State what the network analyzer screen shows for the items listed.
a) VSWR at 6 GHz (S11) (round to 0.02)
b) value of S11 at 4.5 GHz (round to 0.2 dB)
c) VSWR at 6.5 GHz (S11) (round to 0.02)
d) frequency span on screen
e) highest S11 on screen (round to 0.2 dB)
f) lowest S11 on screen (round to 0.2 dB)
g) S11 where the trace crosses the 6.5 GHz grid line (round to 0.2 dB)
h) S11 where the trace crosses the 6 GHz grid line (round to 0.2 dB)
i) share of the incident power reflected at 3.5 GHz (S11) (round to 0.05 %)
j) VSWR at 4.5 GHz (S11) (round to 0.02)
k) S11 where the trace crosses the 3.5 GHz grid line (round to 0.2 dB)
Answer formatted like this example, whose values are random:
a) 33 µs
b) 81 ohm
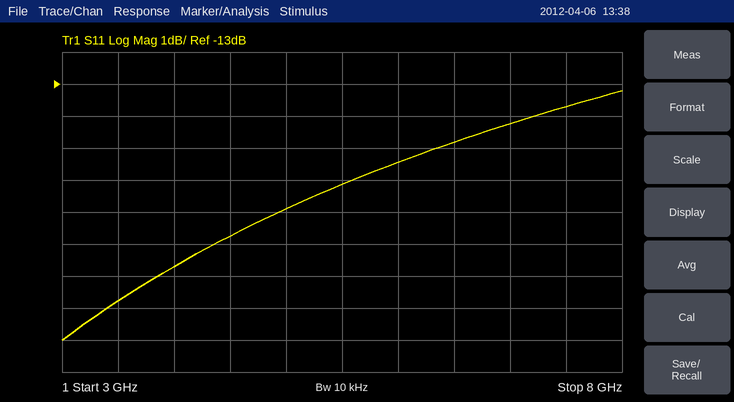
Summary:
a) 1.40
b) -17.8 dB
c) 1.44
d) 5 GHz
e) -13.2 dB
f) -21.0 dB
g) -14.8 dB
h) -15.4 dB
i) 1.05 %
j) 1.30
k) -19.8 dB
